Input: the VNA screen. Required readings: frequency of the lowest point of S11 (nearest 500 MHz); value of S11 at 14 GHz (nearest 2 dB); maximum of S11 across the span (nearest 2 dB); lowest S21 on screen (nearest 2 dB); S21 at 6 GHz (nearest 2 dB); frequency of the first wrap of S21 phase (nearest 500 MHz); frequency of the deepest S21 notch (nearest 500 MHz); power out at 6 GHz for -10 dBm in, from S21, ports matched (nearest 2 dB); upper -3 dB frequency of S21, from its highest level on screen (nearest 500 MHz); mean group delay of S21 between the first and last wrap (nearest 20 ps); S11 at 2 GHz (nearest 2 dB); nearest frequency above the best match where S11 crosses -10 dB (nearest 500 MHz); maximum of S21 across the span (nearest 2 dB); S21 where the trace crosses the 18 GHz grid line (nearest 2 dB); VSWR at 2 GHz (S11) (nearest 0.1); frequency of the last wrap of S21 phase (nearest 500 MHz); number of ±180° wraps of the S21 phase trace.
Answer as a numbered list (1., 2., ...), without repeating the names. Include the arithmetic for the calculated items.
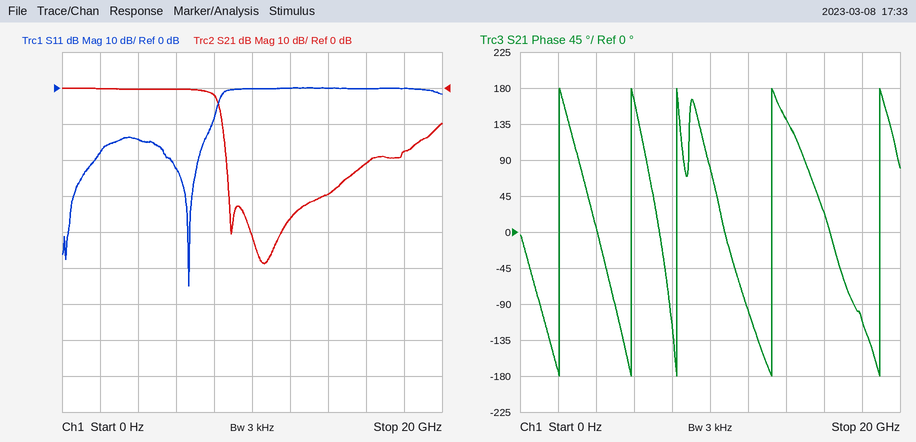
1. 6.5 GHz
2. 0 dB
3. 0 dB
4. -48 dB
5. 0 dB
6. 2.0 GHz
7. 10.5 GHz
8. -10 dBm + (0 dB) = -10 dBm
9. 8.0 GHz
10. 4 cycles / (19.0 GHz − 2.0 GHz) ≈ 235 ps, so 240 ps to the nearest 20 ps
11. -18 dB
12. 8.0 GHz
13. 0 dB
14. -18 dB
15. |Γ| = 10^(-18/20) = 0.1259; VSWR = (1 + 0.1259)/(1 − 0.1259) ≈ 1.3
16. 19.0 GHz
17. 5
